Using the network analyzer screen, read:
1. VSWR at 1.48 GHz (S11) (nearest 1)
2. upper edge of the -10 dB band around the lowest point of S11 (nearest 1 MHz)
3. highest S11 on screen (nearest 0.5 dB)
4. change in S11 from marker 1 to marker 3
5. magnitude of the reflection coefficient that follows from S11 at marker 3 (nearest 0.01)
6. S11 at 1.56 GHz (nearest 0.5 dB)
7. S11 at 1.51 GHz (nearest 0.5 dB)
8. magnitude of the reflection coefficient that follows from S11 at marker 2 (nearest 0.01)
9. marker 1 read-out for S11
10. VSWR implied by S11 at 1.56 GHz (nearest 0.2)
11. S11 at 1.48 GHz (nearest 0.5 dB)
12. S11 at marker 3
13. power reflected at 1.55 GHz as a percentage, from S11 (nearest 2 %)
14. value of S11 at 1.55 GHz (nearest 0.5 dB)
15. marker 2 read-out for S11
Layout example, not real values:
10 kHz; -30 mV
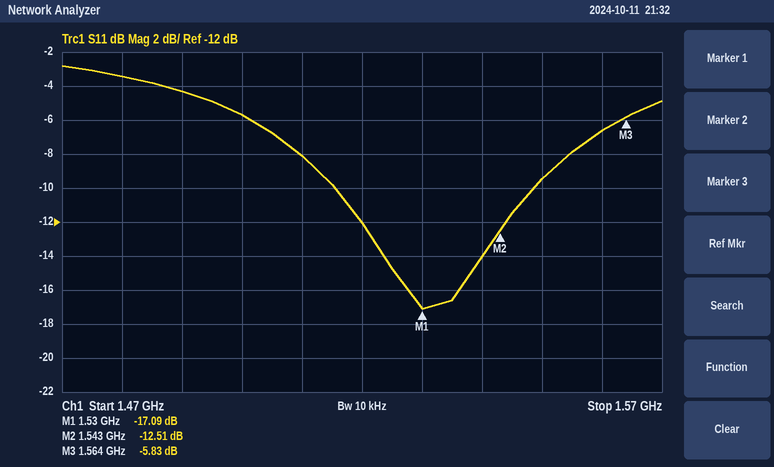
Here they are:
5; 1.549 GHz; -3.0 dB; 11.26 dB; 0.51; -6.5 dB; -8.0 dB; 0.24; -17.09 dB; 2.8; -3.5 dB; -5.83 dB; 12 %; -9.5 dB; -12.51 dB
